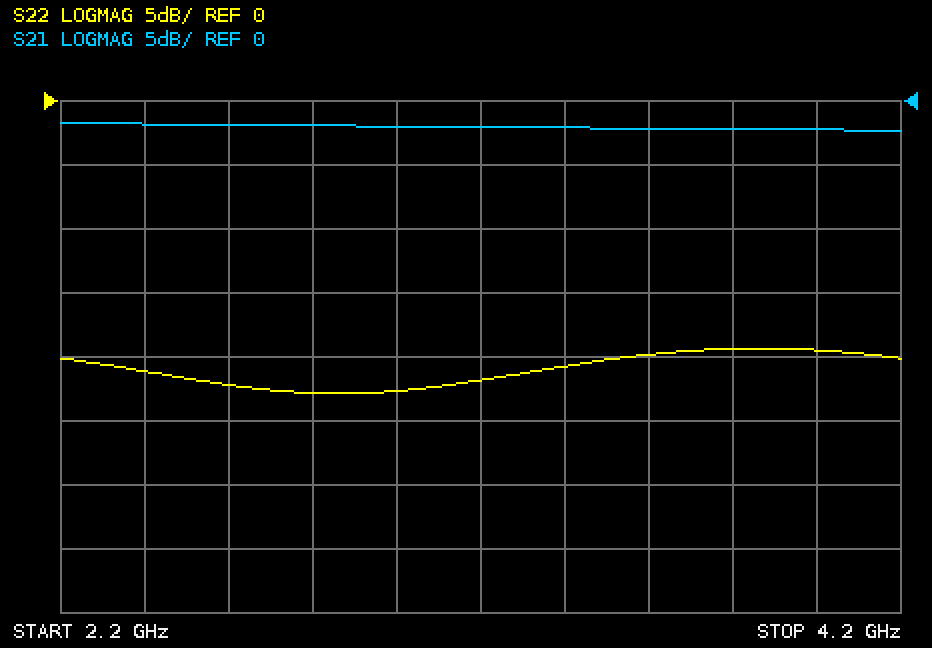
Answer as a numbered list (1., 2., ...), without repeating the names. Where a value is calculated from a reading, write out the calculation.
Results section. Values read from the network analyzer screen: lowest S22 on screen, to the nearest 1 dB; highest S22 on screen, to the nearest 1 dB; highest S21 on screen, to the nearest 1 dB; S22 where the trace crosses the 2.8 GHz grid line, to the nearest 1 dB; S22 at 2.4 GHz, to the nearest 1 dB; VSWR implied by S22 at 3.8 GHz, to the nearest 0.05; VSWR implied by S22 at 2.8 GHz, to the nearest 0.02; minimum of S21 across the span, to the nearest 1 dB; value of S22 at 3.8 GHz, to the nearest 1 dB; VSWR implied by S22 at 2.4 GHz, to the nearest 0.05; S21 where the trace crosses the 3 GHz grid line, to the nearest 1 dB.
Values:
1. -23 dB
2. -19 dB
3. -2 dB
4. -23 dB
5. -21 dB
6. |Γ| = 10^(-19/20) = 0.1122; VSWR = (1 + 0.1122)/(1 − 0.1122) ≈ 1.25
7. |Γ| = 10^(-23/20) = 0.0708; VSWR = (1 + 0.0708)/(1 − 0.0708) ≈ 1.15, so 1.16 to the nearest 0.02
8. -2 dB
9. -19 dB
10. |Γ| = 10^(-21/20) = 0.0891; VSWR = (1 + 0.0891)/(1 − 0.0891) ≈ 1.20
11. -2 dB
